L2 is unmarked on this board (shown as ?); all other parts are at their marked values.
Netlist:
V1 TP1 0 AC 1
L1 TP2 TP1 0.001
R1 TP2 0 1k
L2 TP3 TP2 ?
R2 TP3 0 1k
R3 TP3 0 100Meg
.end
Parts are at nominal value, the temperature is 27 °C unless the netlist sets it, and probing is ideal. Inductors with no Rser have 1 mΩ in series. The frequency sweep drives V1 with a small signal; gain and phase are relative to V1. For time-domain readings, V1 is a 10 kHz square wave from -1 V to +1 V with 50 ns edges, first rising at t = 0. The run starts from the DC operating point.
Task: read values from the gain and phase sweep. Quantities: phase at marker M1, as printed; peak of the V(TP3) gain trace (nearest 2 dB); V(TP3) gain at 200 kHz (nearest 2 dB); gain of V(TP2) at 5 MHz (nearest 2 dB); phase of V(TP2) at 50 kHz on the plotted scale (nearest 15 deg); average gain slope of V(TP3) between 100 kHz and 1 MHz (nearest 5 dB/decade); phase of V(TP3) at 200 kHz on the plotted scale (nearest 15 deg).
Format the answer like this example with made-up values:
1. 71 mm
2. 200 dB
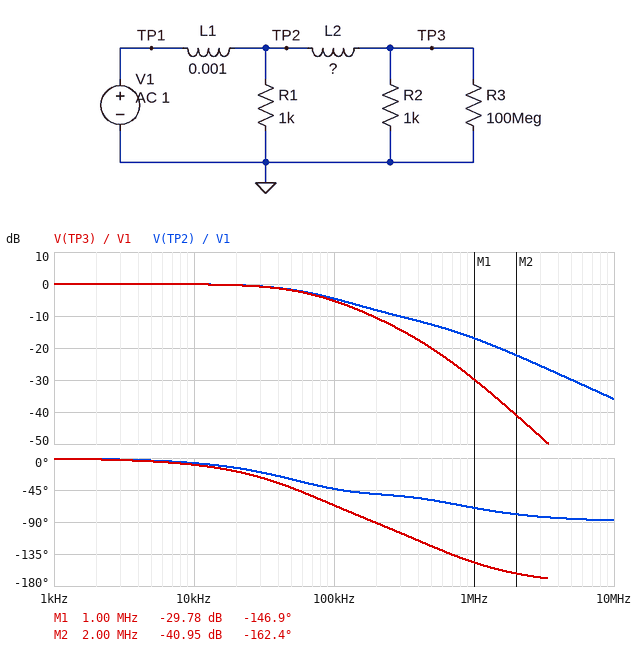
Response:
1. -146.9 deg
2. 0 dB
3. -10 dB
4. -30 dB
5. -30 deg
6. -25 dB/decade
7. -90 deg
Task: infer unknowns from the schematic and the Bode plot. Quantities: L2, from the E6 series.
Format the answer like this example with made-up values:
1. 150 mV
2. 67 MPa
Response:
1. 680 µH
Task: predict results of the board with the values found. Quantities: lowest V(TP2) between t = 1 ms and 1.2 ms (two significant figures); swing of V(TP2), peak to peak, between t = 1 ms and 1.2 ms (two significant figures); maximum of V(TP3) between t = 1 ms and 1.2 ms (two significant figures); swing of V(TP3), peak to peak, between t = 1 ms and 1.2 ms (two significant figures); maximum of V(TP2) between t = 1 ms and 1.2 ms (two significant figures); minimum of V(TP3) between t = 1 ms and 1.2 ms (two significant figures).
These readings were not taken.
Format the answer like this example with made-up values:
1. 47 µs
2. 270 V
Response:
1. -1.0 V
2. 2.0 V
3. 1.0 V
4. 2.0 V
5. 1.0 V
6. -1.0 V
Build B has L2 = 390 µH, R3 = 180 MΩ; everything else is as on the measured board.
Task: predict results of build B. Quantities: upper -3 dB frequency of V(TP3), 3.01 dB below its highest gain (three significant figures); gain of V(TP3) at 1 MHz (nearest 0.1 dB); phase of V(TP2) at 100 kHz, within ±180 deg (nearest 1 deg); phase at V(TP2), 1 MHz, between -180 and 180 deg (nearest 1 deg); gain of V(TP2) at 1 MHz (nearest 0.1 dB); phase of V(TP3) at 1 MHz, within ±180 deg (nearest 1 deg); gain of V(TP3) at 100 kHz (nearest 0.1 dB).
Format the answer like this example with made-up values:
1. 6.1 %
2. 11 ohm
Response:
1. 71.4 kHz
2. -26.4 dB
3. -47 deg
4. -66 deg
5. -17.9 dB
6. -134 deg
7. -4.7 dB
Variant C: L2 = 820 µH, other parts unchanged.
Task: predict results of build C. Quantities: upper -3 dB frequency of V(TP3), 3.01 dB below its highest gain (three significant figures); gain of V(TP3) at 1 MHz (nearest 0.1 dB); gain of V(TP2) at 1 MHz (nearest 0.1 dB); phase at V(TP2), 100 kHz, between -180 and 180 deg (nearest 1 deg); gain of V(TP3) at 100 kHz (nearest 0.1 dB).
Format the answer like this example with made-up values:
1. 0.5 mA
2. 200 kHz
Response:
1. 62.8 kHz
2. -31.1 dB
3. -16.7 dB
4. -42 deg
5. -5.6 dB
